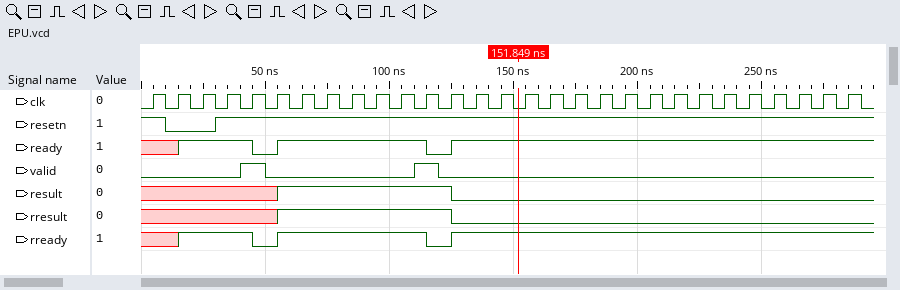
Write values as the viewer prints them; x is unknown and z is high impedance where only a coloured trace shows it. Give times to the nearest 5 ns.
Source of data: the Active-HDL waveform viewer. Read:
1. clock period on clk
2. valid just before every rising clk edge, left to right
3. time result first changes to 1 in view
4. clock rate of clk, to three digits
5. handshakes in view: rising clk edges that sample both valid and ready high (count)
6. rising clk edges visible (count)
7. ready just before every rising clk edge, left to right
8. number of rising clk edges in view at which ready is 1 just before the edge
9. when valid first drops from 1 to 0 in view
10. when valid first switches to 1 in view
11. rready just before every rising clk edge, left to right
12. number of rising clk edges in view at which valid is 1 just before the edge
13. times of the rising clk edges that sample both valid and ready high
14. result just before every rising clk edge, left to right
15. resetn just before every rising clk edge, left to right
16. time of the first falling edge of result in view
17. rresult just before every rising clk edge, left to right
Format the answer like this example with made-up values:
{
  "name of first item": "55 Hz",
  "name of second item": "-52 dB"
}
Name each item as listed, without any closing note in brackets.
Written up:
{
  "clock period on clk": "10 ns",
  "valid just before every rising clk edge, left to right": "0 0 0 0 1 0 0 0 0 0 0 1 0 0 0 0 0 0 0 0 0 0 0 0 0 0 0 0 0",
  "time result first changes to 1 in view": "55 ns",
  "clock rate of clk, to three digits": "100 MHz",
  "handshakes in view: rising clk edges that sample both valid and ready high": "2",
  "rising clk edges visible": "29",
  "ready just before every rising clk edge, left to right": "x x 1 1 1 0 1 1 1 1 1 1 0 1 1 1 1 1 1 1 1 1 1 1 1 1 1 1 1",
  "number of rising clk edges in view at which ready is 1 just before the edge": "25",
  "when valid first drops from 1 to 0 in view": "50 ns",
  "when valid first switches to 1 in view": "40 ns",
  "rready just before every rising clk edge, left to right": "x x 1 1 1 0 1 1 1 1 1 1 0 1 1 1 1 1 1 1 1 1 1 1 1 1 1 1 1",
  "number of rising clk edges in view at which valid is 1 just before the edge": "2",
  "times of the rising clk edges that sample both valid and ready high": "45 ns, 115 ns",
  "result just before every rising clk edge, left to right": "x x x x x x 1 1 1 1 1 1 1 0 0 0 0 0 0 0 0 0 0 0 0 0 0 0 0",
  "resetn just before every rising clk edge, left to right": "1 0 0 1 1 1 1 1 1 1 1 1 1 1 1 1 1 1 1 1 1 1 1 1 1 1 1 1 1",
  "time of the first falling edge of result in view": "125 ns",
  "rresult just before every rising clk edge, left to right": "x x x x x x 1 1 1 1 1 1 1 0 0 0 0 0 0 0 0 0 0 0 0 0 0 0 0"
}
